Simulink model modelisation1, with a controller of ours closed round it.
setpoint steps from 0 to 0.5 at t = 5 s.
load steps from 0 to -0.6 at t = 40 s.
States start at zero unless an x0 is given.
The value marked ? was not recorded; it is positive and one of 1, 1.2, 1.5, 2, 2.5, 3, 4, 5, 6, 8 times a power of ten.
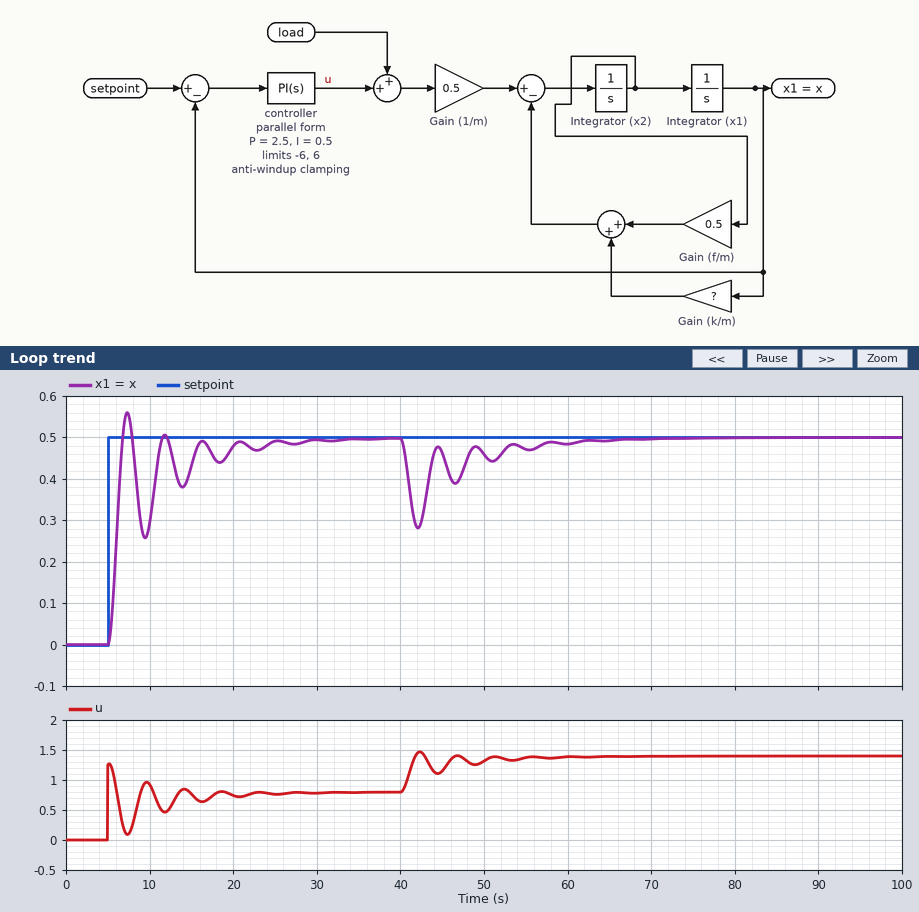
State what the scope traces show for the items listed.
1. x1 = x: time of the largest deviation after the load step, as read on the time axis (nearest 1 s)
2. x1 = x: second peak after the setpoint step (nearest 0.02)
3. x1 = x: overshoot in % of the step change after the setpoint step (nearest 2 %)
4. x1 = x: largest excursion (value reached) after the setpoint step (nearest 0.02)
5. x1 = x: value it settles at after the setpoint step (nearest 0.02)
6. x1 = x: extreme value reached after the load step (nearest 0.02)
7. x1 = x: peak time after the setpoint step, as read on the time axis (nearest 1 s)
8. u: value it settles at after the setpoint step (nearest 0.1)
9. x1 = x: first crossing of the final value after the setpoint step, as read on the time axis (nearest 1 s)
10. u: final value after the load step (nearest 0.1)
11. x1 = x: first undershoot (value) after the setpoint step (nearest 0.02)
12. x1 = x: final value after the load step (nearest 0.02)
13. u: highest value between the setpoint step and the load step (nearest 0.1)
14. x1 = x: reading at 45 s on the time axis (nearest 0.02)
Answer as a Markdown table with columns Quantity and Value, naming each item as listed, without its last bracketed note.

| Quantity | Value |
|---|---|
| x1 = x: time of the largest deviation after the load step, as read on the time axis | 42 s |
| x1 = x: second peak after the setpoint step | 0.50 |
| x1 = x: overshoot in % of the step change after the setpoint step | 12 % |
| x1 = x: largest excursion (value reached) after the setpoint step | 0.56 |
| x1 = x: value it settles at after the setpoint step | 0.50 |
| x1 = x: extreme value reached after the load step | 0.28 |
| x1 = x: peak time after the setpoint step, as read on the time axis | 7 s |
| u: value it settles at after the setpoint step | 0.8 |
| x1 = x: first crossing of the final value after the setpoint step, as read on the time axis | 7 s |
| u: final value after the load step | 1.4 |
| x1 = x: first undershoot (value) after the setpoint step | 0.26 |
| x1 = x: final value after the load step | 0.50 |
| u: highest value between the setpoint step and the load step | 1.3 |
| x1 = x: reading at 45 s on the time axis | 0.46 |
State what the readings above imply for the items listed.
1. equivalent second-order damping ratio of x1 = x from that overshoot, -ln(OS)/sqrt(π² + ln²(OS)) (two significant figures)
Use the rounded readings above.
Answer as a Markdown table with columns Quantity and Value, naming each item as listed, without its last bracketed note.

| Quantity | Value |
|---|---|
| equivalent second-order damping ratio of x1 = x from that overshoot, -ln(OS)/sqrt(π² + ln²(OS)) | 0.56 |
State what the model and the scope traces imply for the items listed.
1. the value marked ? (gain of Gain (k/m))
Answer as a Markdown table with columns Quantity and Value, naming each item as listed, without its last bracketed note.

| Quantity | Value |
|---|---|
| the value marked ? (gain of Gain (k/m)) | 0.8 |
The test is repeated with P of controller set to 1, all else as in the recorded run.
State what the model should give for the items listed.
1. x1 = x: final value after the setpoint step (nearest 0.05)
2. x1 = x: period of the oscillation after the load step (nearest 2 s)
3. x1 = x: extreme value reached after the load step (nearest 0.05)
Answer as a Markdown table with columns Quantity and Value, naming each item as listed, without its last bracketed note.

| Quantity | Value |
|---|---|
| x1 = x: final value after the setpoint step | 0.50 |
| x1 = x: period of the oscillation after the load step | 6 s |
| x1 = x: extreme value reached after the load step | 0.20 |
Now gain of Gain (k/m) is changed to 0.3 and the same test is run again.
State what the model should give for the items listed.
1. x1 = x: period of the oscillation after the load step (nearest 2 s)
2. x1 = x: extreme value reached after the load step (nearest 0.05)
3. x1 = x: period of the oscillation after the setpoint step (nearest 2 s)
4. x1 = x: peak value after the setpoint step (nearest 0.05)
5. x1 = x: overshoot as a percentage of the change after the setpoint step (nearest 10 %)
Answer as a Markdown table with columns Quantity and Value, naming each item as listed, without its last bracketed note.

| Quantity | Value |
|---|---|
| x1 = x: period of the oscillation after the load step | 6 s |
| x1 = x: extreme value reached after the load step | 0.25 |
| x1 = x: period of the oscillation after the setpoint step | 6 s |
| x1 = x: peak value after the setpoint step | 0.70 |
| x1 = x: overshoot as a percentage of the change after the setpoint step | 40 % |
